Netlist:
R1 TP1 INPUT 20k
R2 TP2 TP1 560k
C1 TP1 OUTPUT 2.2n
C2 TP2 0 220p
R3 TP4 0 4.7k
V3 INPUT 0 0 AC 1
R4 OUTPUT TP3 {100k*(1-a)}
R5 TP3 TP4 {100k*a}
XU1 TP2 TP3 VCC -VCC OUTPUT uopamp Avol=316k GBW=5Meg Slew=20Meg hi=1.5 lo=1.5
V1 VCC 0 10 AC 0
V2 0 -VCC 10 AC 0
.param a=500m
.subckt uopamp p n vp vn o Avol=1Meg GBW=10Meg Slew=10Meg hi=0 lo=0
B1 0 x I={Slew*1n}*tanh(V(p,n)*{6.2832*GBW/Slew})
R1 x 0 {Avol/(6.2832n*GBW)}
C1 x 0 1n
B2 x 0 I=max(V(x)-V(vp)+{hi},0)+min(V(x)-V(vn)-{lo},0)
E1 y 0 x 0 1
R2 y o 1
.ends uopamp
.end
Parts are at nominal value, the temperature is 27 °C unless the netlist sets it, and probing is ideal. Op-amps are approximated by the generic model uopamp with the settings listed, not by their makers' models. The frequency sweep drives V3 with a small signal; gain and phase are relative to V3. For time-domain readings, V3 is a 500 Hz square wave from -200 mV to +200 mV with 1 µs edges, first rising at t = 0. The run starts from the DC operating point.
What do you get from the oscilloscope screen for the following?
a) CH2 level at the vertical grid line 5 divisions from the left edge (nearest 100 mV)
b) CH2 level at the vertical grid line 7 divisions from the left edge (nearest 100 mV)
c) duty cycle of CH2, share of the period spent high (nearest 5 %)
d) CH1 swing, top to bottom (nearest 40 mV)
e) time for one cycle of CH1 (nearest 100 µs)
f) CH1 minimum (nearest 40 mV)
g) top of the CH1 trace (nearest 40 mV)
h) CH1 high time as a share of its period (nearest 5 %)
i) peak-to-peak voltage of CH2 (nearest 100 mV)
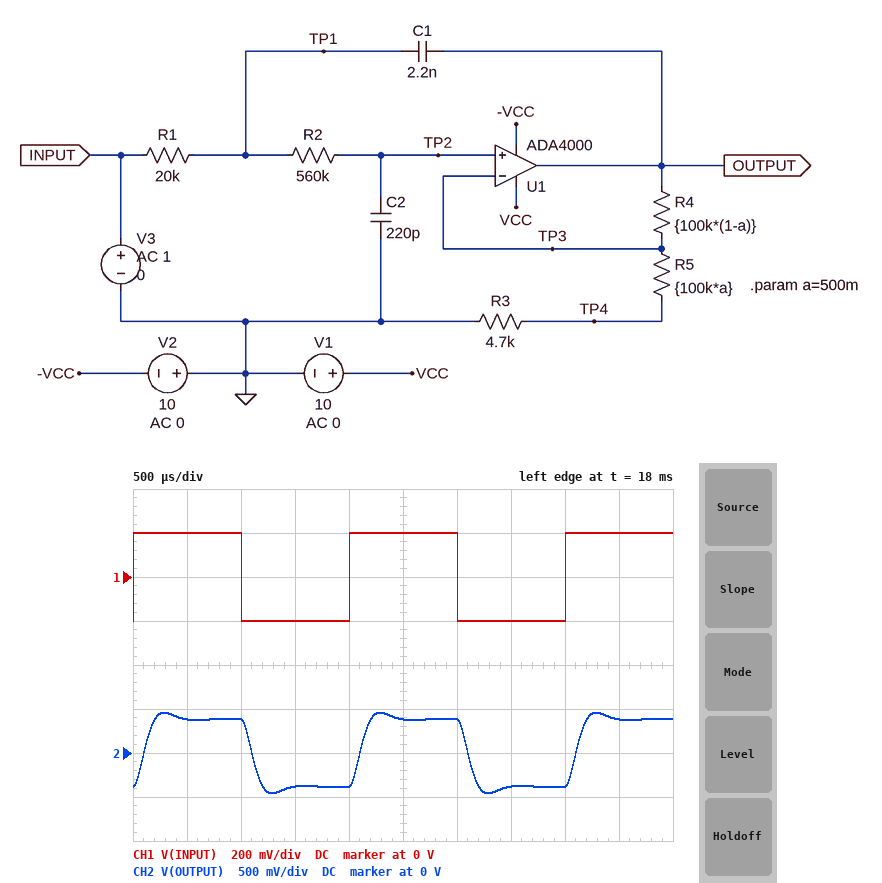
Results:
400 mV
-400 mV
50 %
400 mV
2.0 ms
-200 mV
200 mV
50 %
900 mV
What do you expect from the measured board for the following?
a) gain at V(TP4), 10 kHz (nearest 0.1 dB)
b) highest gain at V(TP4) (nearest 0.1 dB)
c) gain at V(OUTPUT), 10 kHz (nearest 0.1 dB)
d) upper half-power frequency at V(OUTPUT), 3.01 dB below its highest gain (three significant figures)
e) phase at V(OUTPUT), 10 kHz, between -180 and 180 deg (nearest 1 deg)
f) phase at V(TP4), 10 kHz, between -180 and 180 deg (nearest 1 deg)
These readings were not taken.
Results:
-47.8 dB
-20.9 dB
-20.9 dB
2.42 kHz
-165 deg
-165 deg
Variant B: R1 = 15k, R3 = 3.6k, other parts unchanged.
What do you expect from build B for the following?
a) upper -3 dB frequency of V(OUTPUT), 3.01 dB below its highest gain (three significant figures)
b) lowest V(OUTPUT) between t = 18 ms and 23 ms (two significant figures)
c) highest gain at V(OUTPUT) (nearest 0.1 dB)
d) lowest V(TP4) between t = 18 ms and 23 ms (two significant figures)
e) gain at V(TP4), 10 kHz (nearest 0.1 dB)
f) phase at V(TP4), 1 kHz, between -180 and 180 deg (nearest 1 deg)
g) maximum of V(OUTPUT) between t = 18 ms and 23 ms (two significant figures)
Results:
2.34 kHz
-410 mV
5.7 dB
-14 mV
-47.7 dB
-36 deg
410 mV
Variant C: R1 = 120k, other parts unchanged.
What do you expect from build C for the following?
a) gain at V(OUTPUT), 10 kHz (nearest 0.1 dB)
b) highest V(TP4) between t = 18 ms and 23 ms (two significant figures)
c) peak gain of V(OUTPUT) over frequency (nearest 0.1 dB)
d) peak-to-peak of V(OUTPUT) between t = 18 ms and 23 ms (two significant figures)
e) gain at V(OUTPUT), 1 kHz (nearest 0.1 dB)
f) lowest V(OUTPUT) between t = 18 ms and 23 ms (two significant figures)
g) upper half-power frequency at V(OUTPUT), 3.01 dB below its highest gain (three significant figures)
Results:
-36.5 dB
380 mV
11.8 dB
17 V
9.5 dB
-8.5 V
1.03 kHz
